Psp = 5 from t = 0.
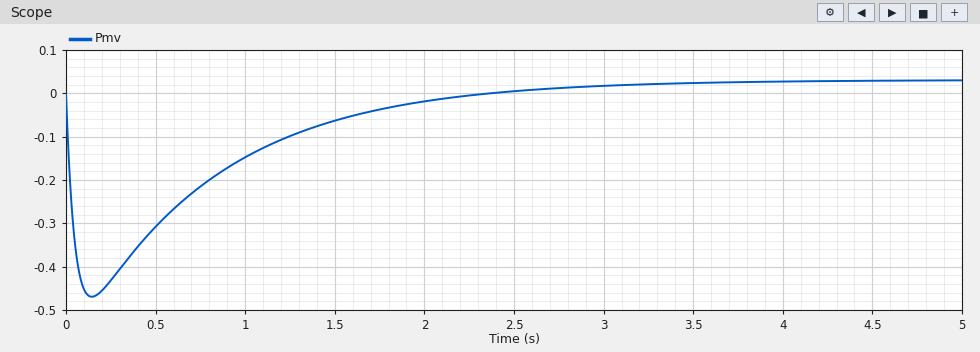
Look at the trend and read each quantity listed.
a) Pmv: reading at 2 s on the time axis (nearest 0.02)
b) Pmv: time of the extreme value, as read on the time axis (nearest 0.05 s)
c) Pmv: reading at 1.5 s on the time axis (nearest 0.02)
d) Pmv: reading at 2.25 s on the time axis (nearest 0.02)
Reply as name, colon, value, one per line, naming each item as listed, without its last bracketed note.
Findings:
Pmv: reading at 2 s on the time axis: -0.02
Pmv: time of the extreme value, as read on the time axis: 0.15 s
Pmv: reading at 1.5 s on the time axis: -0.06
Pmv: reading at 2.25 s on the time axis: 0.00
